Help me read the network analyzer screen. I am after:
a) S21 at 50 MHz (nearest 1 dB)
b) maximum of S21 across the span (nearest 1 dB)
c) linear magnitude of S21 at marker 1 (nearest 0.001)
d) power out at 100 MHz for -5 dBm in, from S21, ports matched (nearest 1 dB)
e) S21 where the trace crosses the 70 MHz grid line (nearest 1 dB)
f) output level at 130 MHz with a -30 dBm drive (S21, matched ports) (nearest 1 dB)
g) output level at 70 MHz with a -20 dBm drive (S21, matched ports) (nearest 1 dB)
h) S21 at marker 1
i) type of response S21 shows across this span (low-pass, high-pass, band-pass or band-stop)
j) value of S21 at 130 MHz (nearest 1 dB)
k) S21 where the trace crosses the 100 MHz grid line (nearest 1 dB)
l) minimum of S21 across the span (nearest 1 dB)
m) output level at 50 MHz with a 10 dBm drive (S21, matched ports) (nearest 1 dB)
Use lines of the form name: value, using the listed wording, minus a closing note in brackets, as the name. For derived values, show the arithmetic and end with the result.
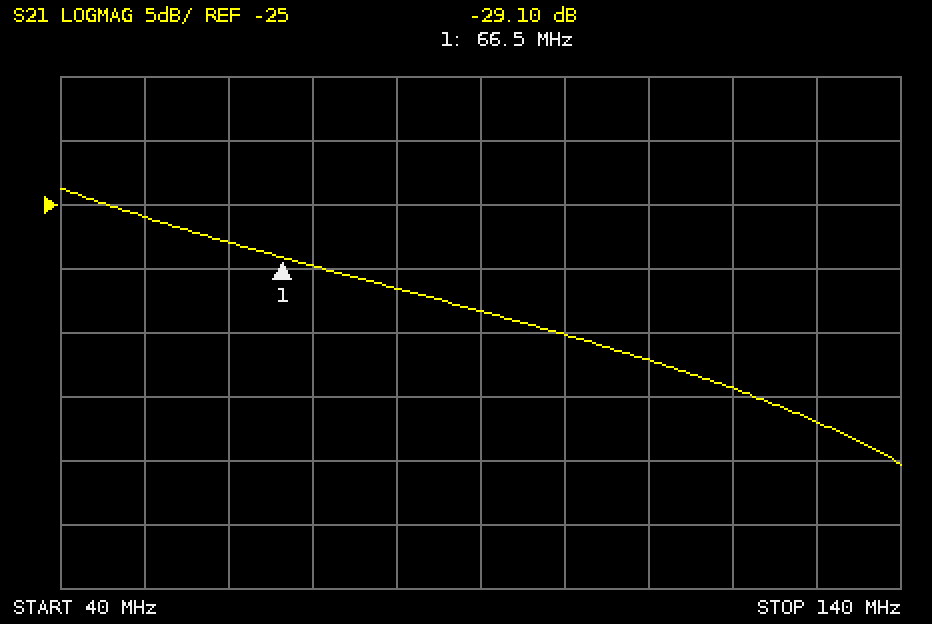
S21 at 50 MHz: -26 dB
maximum of S21 across the span: -24 dB
linear magnitude of S21 at marker 1: 10^(-29.1/20) ≈ 0.035
power out at 100 MHz for -5 dBm in, from S21, ports matched: -5 dBm + (-35 dB) = -40 dBm
S21 where the trace crosses the 70 MHz grid line: -30 dB
output level at 130 MHz with a -30 dBm drive (S21, matched ports): -30 dBm + (-42 dB) = -72 dBm
output level at 70 MHz with a -20 dBm drive (S21, matched ports): -20 dBm + (-30 dB) = -50 dBm
S21 at marker 1: -29.10 dB
type of response S21 shows across this span: low-pass
value of S21 at 130 MHz: -42 dB
S21 where the trace crosses the 100 MHz grid line: -35 dB
minimum of S21 across the span: -45 dB
output level at 50 MHz with a 10 dBm drive (S21, matched ports): 10 dBm + (-26 dB) = -16 dBm
